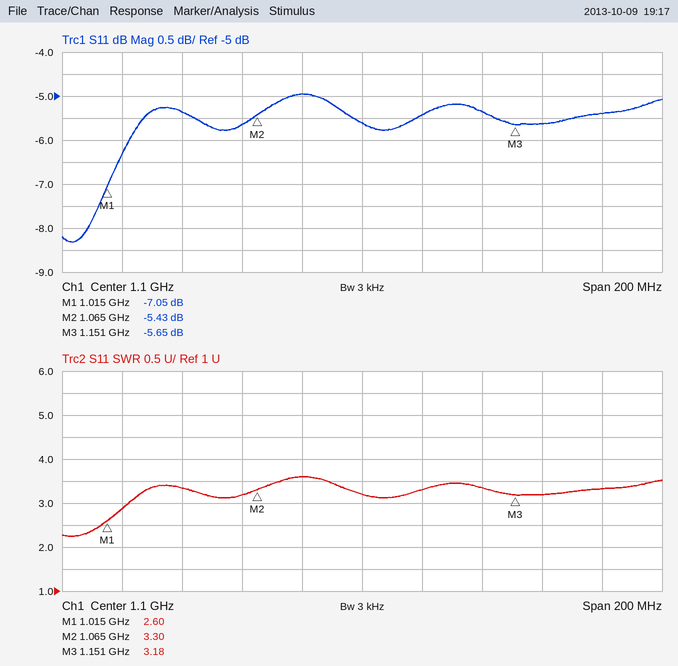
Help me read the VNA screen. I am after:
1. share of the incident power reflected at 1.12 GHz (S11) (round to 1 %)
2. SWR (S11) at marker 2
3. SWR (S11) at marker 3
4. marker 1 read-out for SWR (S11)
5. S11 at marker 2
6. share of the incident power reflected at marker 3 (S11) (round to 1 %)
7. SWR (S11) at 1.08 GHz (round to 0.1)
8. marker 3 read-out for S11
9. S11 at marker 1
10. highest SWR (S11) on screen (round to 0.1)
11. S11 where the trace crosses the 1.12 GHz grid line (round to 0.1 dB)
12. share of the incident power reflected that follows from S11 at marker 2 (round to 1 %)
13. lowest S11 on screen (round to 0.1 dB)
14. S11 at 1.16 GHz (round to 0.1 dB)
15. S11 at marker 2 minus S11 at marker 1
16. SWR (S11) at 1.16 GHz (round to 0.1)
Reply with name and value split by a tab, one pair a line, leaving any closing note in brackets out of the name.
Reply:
share of the incident power reflected at 1.12 GHz (S11)	29 %
SWR (S11) at marker 2	3.30
SWR (S11) at marker 3	3.18
marker 1 read-out for SWR	2.60
S11 at marker 2	-5.43 dB
share of the incident power reflected at marker 3 (S11)	27 %
SWR (S11) at 1.08 GHz	3.6
marker 3 read-out for S11	-5.65 dB
S11 at marker 1	-7.05 dB
highest SWR (S11) on screen	3.6
S11 where the trace crosses the 1.12 GHz grid line	-5.4 dB
share of the incident power reflected that follows from S11 at marker 2	29 %
lowest S11 on screen	-8.3 dB
S11 at 1.16 GHz	-5.6 dB
S11 at marker 2 minus S11 at marker 1	1.62 dB
SWR (S11) at 1.16 GHz	3.2
